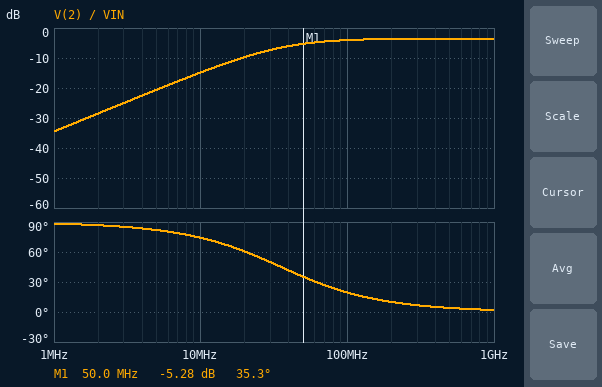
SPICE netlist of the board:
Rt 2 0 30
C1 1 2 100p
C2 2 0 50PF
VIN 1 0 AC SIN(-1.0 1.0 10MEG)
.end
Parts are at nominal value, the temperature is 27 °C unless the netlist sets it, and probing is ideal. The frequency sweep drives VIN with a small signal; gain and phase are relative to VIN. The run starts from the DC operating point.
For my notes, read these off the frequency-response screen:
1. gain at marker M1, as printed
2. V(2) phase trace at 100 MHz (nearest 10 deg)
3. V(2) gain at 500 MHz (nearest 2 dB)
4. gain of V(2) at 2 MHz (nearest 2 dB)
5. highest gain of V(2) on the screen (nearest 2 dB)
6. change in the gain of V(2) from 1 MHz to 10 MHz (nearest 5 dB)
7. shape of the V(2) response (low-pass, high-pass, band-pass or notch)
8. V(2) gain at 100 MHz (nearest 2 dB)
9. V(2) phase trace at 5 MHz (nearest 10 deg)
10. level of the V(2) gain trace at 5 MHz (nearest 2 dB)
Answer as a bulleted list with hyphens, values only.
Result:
- -5.28 dB
- 20 deg
- -4 dB
- -28 dB
- -4 dB
- 20 dB
- high-pass
- -4 dB
- 80 deg
- -20 dB
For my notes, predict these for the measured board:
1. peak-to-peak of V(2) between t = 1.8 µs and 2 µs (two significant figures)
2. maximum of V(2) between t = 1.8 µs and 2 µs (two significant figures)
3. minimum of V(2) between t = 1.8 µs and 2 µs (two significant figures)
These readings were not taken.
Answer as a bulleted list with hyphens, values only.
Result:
- 360 mV
- 180 mV
- -180 mV
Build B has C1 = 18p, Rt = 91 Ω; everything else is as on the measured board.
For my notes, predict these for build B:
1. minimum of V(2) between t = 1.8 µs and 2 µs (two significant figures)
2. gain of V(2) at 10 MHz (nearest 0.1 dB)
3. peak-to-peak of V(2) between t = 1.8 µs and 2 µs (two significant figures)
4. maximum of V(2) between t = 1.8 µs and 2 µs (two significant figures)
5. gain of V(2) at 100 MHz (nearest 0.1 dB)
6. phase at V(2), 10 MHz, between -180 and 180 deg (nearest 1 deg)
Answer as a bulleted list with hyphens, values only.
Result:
- -96 mV
- -20.4 dB
- 190 mV
- 96 mV
- -11.8 dB
- 69 deg
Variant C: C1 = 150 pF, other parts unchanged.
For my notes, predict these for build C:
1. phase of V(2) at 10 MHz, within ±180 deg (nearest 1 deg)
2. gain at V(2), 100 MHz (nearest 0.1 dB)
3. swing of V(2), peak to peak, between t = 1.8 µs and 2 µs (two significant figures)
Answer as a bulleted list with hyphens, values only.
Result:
- 69 deg
- -2.8 dB
- 530 mV
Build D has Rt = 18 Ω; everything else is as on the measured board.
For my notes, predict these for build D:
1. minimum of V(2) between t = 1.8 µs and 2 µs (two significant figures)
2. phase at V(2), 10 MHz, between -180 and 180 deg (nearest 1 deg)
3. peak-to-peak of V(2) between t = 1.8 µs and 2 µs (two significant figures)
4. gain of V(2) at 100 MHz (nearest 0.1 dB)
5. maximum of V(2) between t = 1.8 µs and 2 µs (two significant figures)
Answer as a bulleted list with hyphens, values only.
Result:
- -110 mV
- 80 deg
- 220 mV
- -4.8 dB
- 110 mV
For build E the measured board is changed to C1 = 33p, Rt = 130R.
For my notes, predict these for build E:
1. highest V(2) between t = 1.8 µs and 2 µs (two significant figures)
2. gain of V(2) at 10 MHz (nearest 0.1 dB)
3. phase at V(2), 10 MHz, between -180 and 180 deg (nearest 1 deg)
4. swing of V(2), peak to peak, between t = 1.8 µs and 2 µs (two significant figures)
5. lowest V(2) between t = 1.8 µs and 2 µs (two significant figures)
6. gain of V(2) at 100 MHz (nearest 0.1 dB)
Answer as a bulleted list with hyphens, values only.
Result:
- 220 mV
- -13.0 dB
- 56 deg
- 450 mV
- -220 mV
- -8.1 dB
